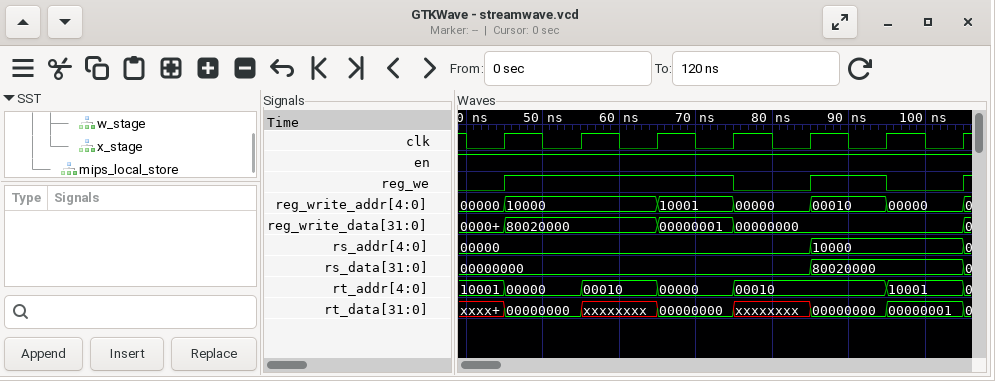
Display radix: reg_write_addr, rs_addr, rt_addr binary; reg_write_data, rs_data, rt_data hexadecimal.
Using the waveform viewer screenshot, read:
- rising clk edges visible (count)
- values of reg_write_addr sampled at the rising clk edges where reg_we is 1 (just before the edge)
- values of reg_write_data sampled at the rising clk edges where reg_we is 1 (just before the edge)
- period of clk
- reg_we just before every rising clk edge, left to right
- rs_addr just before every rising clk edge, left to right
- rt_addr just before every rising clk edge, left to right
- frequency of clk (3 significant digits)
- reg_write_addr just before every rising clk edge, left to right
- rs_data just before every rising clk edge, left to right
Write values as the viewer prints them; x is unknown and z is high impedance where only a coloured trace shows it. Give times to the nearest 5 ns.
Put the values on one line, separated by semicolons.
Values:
7; 10000, 10000, 10001, 00010; 80020000, 80020000, 00000001, 00000000; 10 ns; 0 1 1 1 0 1 0; 00000, 00000, 00000, 00000, 00000, 10000, 10000; 10001, 00000, 00010, 00000, 00010, 00010, 10001; 100 MHz; 00000, 10000, 10000, 10001, 00000, 00010, 00000; 00000000, 00000000, 00000000, 00000000, 00000000, 80020000, 80020000
